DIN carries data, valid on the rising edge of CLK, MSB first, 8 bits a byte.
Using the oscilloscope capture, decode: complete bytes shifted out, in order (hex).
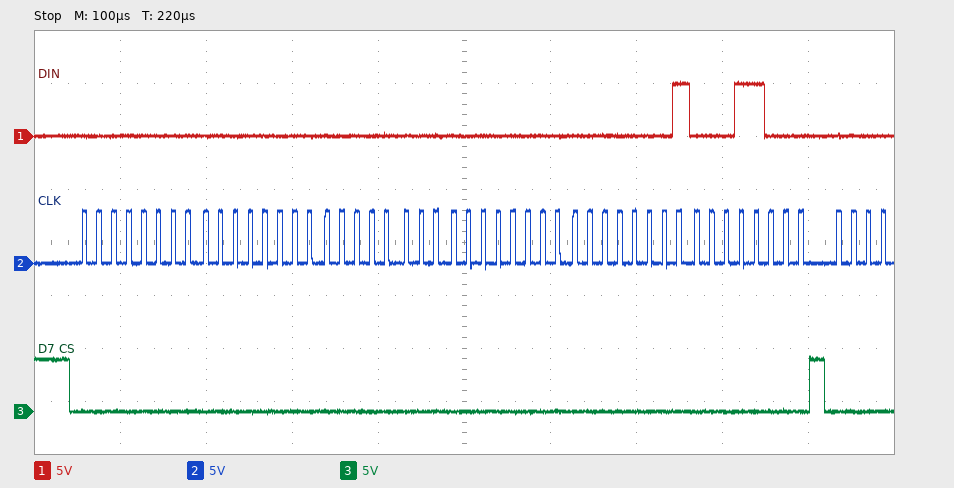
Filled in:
00 00 00 00 01 18
